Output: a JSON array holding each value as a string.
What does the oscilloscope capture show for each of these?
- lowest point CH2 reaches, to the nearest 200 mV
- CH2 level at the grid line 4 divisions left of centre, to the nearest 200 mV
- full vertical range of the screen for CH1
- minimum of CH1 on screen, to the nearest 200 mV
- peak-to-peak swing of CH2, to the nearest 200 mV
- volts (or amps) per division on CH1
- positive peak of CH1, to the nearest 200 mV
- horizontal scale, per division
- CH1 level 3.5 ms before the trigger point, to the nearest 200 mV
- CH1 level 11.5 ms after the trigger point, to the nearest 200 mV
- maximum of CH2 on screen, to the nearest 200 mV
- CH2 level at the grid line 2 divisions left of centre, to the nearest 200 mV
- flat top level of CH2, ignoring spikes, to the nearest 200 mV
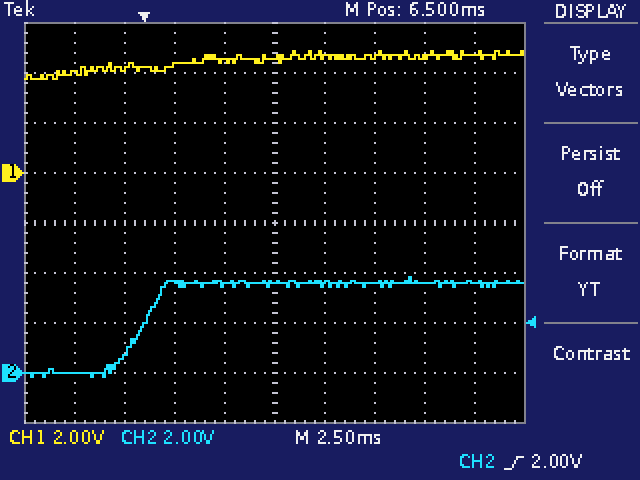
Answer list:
["-200 mV", "0.0 V", "16 V", "3.8 V", "4.0 V", "2 V", "4.8 V", "2.5 ms", "4.0 V", "4.6 V", "3.8 V", "3.6 V", "3.6 V"]
